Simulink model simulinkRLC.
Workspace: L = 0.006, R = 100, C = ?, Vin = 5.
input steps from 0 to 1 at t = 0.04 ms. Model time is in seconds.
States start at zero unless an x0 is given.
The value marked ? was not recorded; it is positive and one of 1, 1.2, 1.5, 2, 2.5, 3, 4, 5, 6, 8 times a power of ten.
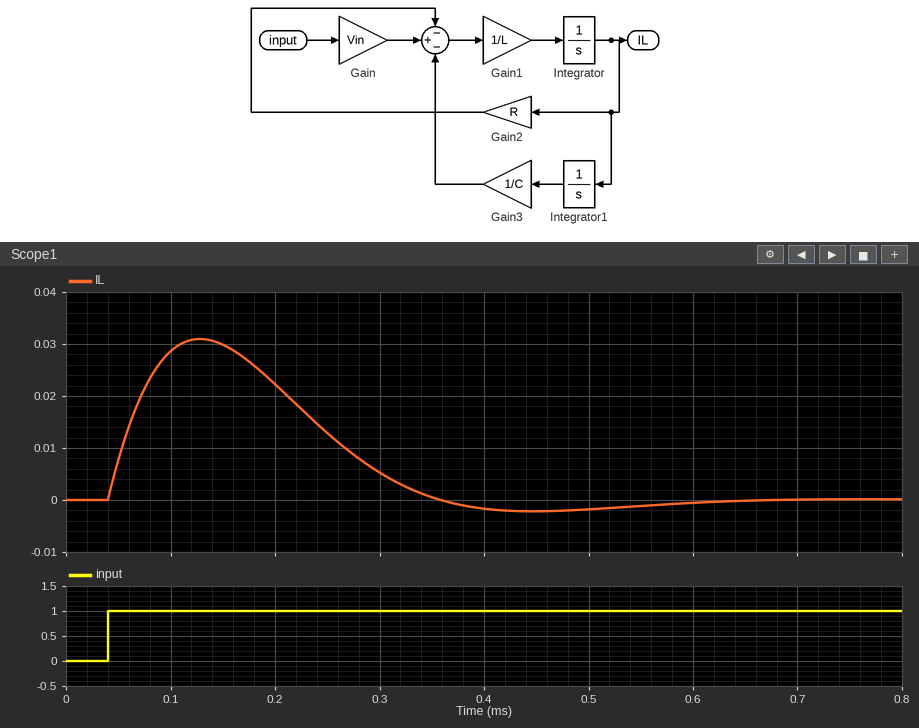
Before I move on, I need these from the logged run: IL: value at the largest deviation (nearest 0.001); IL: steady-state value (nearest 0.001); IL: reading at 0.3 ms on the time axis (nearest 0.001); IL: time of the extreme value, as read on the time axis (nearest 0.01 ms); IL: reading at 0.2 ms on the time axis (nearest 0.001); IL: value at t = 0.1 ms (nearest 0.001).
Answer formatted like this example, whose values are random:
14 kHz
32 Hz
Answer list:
0.031
0.000
0.005
0.13 ms
0.022
0.029
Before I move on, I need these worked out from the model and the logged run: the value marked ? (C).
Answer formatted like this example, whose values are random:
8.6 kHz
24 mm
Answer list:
1e-06
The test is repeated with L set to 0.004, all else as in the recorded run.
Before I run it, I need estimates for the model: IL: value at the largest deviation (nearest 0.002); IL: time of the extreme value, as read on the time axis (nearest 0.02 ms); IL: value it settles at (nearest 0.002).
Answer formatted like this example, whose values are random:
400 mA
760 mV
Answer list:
0.034
0.10 ms
0.000
